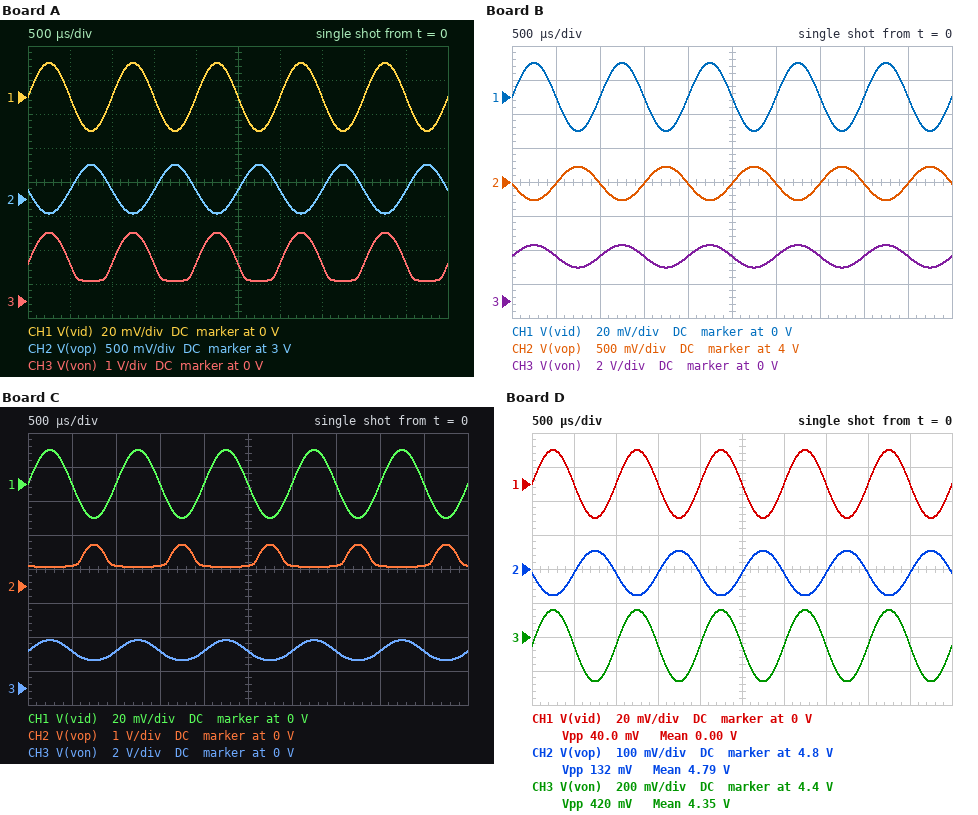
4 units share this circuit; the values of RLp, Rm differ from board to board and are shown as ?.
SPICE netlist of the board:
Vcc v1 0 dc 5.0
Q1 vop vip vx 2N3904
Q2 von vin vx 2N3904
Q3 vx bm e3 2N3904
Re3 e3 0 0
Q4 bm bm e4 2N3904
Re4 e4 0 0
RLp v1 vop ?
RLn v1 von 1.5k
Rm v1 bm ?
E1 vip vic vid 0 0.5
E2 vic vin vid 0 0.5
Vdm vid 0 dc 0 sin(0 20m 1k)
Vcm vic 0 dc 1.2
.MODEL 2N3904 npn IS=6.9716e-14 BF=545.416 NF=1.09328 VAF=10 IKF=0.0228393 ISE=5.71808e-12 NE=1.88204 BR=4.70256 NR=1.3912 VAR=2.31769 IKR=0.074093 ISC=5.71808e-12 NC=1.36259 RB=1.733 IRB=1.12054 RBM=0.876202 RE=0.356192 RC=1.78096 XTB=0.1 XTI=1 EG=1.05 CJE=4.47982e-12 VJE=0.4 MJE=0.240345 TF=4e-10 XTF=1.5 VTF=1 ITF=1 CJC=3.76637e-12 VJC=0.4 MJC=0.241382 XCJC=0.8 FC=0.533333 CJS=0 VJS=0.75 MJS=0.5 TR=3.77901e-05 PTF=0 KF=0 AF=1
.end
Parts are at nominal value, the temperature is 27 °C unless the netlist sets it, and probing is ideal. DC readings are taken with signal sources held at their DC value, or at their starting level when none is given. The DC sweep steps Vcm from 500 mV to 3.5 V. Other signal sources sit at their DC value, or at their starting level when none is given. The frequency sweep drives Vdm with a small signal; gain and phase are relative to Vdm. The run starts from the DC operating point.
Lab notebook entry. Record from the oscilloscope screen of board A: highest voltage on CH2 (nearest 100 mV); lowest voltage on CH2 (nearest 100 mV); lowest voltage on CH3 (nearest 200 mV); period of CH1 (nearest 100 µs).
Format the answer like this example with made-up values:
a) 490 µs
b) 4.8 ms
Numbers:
a) 3.5 V
b) 2.8 V
c) 600 mV
d) 1.0 ms
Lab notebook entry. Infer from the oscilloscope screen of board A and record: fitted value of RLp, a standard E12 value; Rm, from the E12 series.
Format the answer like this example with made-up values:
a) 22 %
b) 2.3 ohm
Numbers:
a) 560 Ω
b) 680 Ω
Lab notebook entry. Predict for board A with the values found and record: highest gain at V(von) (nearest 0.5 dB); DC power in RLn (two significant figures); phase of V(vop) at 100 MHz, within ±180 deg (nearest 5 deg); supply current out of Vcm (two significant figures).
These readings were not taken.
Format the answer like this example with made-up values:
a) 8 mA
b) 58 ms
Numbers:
a) 33.0 dB
b) 10 mW
c) 140 deg
d) 38 µA
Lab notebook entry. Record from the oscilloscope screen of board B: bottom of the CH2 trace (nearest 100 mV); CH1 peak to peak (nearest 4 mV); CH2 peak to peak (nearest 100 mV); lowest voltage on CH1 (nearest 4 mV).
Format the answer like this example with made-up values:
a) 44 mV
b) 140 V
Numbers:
a) 3.7 V
b) 40 mV
c) 500 mV
d) -20 mV
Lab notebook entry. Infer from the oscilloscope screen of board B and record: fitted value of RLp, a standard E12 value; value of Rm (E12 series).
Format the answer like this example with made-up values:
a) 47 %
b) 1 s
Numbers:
a) 560 Ω
b) 1.2 kΩ
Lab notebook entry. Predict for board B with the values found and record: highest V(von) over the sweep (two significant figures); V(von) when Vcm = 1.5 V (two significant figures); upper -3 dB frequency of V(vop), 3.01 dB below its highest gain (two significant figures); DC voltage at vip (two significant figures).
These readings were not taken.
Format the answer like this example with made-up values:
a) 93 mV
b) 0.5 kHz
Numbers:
a) 5.0 V
b) 2.5 V
c) 150 MHz
d) 1.2 V
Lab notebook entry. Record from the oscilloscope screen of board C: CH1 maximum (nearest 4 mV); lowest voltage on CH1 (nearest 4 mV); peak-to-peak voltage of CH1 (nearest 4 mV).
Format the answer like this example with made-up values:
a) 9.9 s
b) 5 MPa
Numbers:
a) 20 mV
b) -20 mV
c) 40 mV
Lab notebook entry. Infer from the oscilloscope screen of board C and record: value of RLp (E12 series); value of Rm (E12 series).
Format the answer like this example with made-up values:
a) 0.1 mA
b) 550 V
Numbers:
a) 3.3 kΩ
b) 1.2 kΩ
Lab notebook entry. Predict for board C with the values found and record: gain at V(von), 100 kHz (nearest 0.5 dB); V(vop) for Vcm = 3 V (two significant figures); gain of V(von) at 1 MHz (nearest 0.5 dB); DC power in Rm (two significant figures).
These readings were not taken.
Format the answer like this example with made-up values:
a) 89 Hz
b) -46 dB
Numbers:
a) 30.0 dB
b) 2.3 V
c) 30.0 dB
d) 15 mW
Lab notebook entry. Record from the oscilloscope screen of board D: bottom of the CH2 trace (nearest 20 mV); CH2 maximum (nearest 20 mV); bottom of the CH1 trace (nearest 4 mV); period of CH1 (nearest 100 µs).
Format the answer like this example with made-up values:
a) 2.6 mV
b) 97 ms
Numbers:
a) 4.72 V
b) 4.86 V
c) -20 mV
d) 1.0 ms
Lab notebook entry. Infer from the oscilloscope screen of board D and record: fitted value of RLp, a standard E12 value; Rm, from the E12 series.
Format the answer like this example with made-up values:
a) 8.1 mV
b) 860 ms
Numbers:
a) 470 Ω
b) 4.7 kΩ
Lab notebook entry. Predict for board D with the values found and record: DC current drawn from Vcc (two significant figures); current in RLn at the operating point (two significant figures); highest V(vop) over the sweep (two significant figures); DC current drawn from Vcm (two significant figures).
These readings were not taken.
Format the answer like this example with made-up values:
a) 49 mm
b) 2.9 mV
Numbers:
a) 1.8 mA
b) 430 µA
c) 5.0 V
d) 7.1 µA
